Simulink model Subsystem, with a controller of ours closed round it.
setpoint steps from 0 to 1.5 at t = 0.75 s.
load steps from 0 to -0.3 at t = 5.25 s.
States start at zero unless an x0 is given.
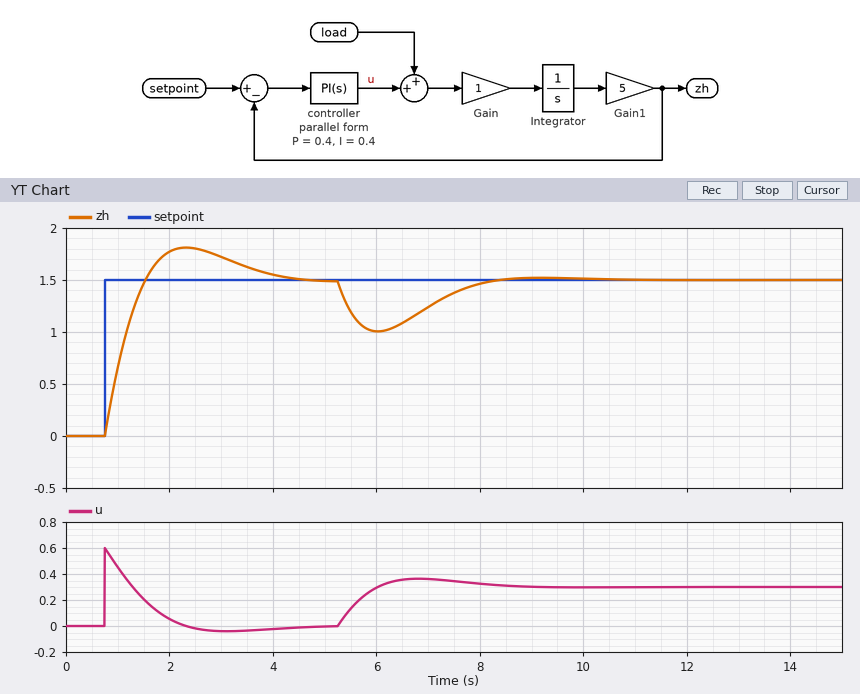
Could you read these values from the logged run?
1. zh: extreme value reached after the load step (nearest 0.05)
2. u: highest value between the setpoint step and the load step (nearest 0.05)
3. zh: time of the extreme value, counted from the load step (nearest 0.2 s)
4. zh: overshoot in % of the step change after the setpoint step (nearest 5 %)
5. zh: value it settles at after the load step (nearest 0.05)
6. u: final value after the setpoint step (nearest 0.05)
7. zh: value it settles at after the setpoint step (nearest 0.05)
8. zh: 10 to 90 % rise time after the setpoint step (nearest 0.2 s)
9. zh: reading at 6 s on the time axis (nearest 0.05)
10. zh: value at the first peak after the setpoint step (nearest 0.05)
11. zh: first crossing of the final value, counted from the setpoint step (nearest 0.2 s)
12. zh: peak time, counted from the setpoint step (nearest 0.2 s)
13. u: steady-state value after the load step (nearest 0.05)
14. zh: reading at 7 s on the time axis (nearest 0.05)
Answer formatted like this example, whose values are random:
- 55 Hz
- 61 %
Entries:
- 1.00
- 0.60
- 0.8 s
- 20 %
- 1.50
- 0.00
- 1.50
- 0.6 s
- 1.00
- 1.80
- 0.8 s
- 1.6 s
- 0.30
- 1.25
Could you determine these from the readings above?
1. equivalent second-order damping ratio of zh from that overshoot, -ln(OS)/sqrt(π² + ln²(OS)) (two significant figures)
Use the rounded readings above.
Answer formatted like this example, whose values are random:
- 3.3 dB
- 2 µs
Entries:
- 0.46
